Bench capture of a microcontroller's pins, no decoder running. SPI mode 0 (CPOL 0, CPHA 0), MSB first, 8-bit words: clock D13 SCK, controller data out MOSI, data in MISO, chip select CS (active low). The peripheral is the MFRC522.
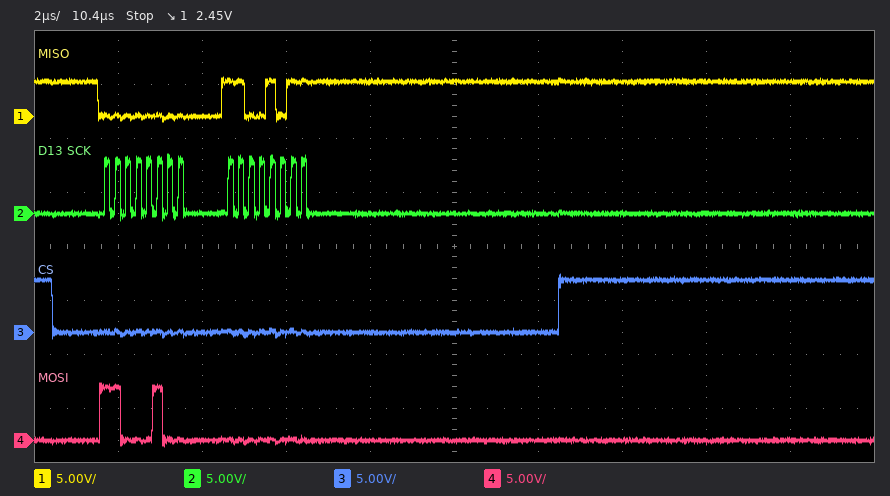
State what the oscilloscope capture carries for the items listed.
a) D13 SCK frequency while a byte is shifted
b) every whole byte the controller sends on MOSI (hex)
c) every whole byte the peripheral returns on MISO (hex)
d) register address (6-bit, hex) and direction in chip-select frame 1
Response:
4 MHz
C4 00
00 CB
0x22 read
